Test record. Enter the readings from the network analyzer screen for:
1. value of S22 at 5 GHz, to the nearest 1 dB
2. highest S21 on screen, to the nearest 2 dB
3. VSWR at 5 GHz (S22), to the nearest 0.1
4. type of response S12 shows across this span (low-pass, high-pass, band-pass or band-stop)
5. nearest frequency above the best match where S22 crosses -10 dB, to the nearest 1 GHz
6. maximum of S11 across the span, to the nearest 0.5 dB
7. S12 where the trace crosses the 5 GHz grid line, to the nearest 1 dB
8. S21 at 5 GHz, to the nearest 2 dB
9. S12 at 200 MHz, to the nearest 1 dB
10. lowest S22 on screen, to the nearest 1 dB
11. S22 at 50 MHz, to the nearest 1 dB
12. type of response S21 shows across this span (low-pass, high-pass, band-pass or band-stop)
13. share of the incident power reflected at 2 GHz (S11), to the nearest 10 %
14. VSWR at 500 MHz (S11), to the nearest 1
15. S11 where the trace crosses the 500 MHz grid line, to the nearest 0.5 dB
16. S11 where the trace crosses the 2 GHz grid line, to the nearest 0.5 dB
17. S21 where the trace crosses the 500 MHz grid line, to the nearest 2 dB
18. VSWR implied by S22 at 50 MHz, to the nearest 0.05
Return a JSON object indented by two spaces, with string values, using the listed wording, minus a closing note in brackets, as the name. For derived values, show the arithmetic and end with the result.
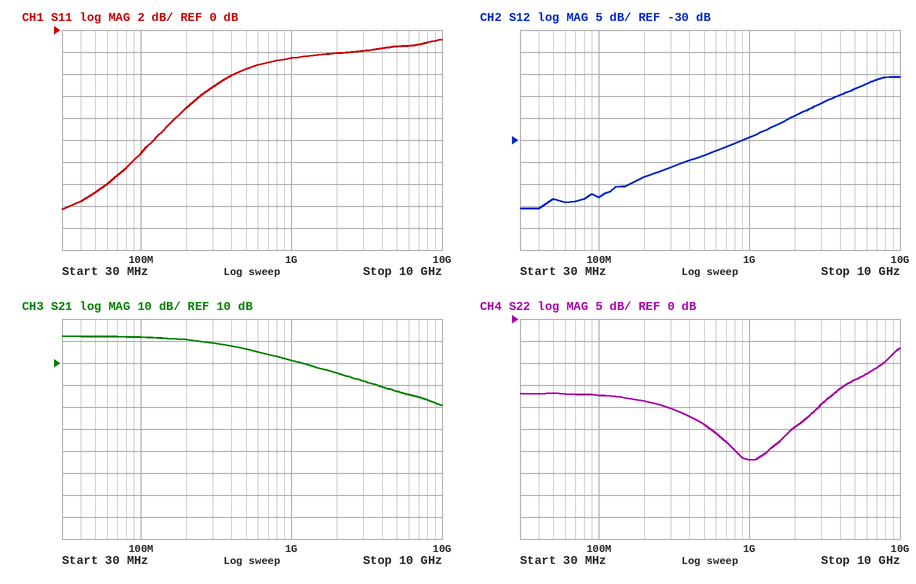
{
  "value of S22 at 5 GHz, to the nearest 1 dB": "-14 dB",
  "highest S21 on screen, to the nearest 2 dB": "22 dB",
  "VSWR at 5 GHz (S22), to the nearest 0.1": "|Γ| = 10^(-14/20) = 0.1995; VSWR = (1 + 0.1995)/(1 − 0.1995) ≈ 1.5",
  "type of response S12 shows across this span": "high-pass",
  "nearest frequency above the best match where S22 crosses -10 dB, to the nearest 1 GHz": "8 GHz",
  "maximum of S11 across the span, to the nearest 0.5 dB": "-1.0 dB",
  "S12 where the trace crosses the 5 GHz grid line, to the nearest 1 dB": "-18 dB",
  "S21 at 5 GHz, to the nearest 2 dB": "-2 dB",
  "S12 at 200 MHz, to the nearest 1 dB": "-38 dB",
  "lowest S22 on screen, to the nearest 1 dB": "-32 dB",
  "S22 at 50 MHz, to the nearest 1 dB": "-17 dB",
  "type of response S21 shows across this span": "low-pass",
  "share of the incident power reflected at 2 GHz (S11), to the nearest 10 %": "10^(-2/10) ≈ 63.1 %, so 60 % to the nearest 10 %",
  "VSWR at 500 MHz (S11), to the nearest 1": "|Γ| = 10^(-3.5/20) = 0.6683; VSWR = (1 + 0.6683)/(1 − 0.6683) ≈ 5",
  "S11 where the trace crosses the 500 MHz grid line, to the nearest 0.5 dB": "-3.5 dB",
  "S11 where the trace crosses the 2 GHz grid line, to the nearest 0.5 dB": "-2.0 dB",
  "S21 where the trace crosses the 500 MHz grid line, to the nearest 2 dB": "16 dB",
  "VSWR implied by S22 at 50 MHz, to the nearest 0.05": "|Γ| = 10^(-17/20) = 0.1413; VSWR = (1 + 0.1413)/(1 − 0.1413) ≈ 1.33, so 1.35 to the nearest 0.05"
}
